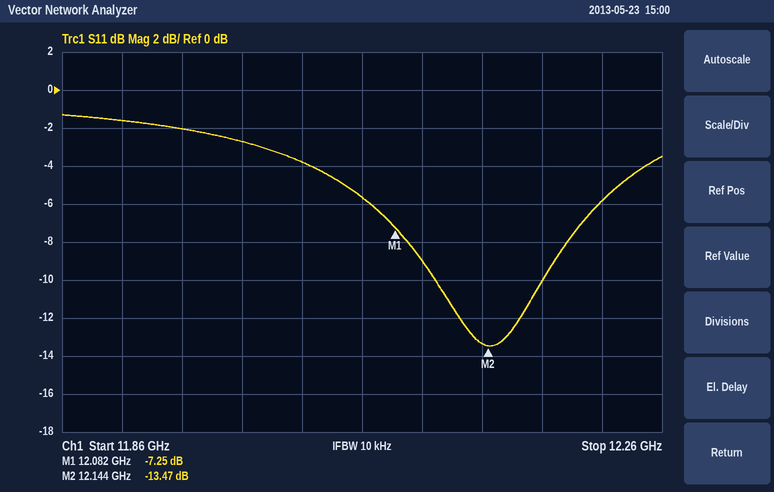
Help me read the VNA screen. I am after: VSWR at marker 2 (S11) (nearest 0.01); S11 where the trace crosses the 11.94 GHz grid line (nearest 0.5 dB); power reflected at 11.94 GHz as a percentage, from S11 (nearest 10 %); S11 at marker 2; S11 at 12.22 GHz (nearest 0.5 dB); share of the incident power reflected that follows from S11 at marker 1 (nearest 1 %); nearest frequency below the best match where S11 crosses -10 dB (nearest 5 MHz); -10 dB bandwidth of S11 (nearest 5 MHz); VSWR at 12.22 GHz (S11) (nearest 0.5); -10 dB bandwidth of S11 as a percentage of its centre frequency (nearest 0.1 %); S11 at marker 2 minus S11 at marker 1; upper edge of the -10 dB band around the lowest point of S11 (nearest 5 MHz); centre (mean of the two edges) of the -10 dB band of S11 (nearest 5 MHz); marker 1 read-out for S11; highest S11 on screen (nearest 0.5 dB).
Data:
1.54
-2.0 dB
60 %
-13.47 dB
-6.0 dB
19 %
12.110 GHz
70 MHz
3.0
0.6 %
-6.22 dB
12.180 GHz
12.145 GHz
-7.25 dB
-1.5 dB
